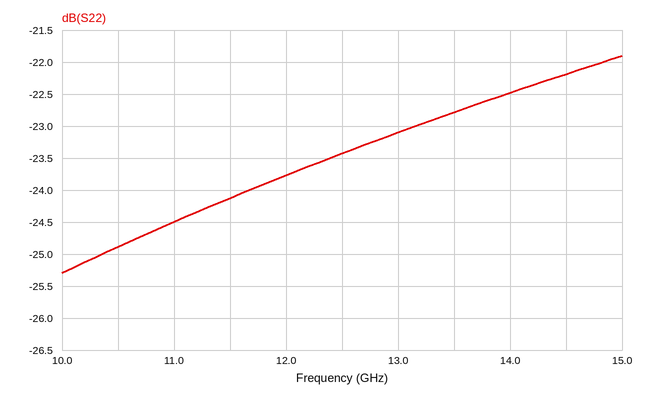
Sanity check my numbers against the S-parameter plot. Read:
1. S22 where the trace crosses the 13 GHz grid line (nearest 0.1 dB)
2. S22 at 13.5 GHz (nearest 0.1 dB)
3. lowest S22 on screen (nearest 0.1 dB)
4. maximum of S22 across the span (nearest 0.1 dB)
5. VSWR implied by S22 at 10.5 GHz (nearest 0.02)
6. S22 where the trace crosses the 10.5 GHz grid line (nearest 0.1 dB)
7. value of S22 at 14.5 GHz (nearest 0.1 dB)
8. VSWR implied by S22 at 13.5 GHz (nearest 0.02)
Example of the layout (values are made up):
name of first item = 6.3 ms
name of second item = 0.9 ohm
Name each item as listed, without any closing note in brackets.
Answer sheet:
S22 where the trace crosses the 13 GHz grid line = -23.1 dB
S22 at 13.5 GHz = -22.8 dB
lowest S22 on screen = -25.3 dB
maximum of S22 across the span = -21.9 dB
VSWR implied by S22 at 10.5 GHz = 1.12
S22 where the trace crosses the 10.5 GHz grid line = -24.9 dB
value of S22 at 14.5 GHz = -22.2 dB
VSWR implied by S22 at 13.5 GHz = 1.16
